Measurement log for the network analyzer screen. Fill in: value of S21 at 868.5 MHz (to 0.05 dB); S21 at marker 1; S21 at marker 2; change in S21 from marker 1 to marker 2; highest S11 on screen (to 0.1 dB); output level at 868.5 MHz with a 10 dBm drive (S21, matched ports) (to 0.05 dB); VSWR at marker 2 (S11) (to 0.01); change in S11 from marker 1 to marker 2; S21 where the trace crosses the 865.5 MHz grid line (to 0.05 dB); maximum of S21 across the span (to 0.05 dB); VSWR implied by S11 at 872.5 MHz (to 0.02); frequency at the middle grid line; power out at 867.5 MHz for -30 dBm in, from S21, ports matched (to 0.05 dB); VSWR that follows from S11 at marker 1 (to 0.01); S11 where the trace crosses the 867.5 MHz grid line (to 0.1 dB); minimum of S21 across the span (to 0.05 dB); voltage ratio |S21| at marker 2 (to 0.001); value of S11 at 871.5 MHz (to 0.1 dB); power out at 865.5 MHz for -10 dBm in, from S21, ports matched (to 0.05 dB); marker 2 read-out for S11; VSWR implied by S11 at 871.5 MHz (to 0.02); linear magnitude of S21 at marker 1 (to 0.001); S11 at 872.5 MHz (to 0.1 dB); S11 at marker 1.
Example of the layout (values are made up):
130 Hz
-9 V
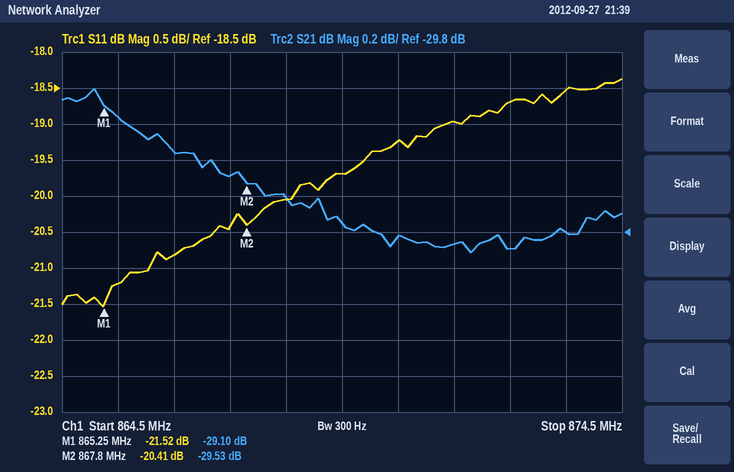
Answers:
-29.60 dB
-29.10 dB
-29.53 dB
-0.43 dB
-18.4 dB
-19.60 dBm
1.21
1.11 dB
-29.15 dB
-29.00 dB
1.26
869.5 MHz
-59.50 dBm
1.18
-20.4 dB
-29.90 dB
0.033
-19.0 dB
-39.15 dBm
-20.41 dB
1.26
0.035
-18.7 dB
-21.52 dB
